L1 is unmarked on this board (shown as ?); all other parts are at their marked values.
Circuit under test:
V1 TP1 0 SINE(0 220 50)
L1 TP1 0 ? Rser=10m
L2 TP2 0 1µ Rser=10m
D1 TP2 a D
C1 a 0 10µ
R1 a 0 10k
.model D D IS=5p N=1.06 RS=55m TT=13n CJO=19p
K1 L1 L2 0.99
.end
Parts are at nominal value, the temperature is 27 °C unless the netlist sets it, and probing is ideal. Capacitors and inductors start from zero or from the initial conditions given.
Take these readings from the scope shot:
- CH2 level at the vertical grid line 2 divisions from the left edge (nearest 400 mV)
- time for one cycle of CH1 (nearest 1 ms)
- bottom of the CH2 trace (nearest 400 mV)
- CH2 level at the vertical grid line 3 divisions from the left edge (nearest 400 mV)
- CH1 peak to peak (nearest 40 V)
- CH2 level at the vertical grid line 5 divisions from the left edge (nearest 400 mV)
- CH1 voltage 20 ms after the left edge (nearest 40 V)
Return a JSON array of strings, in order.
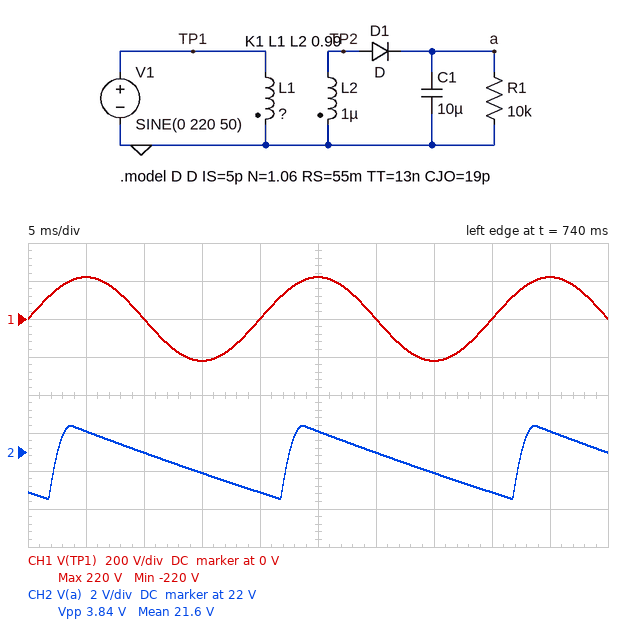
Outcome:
["22.0 V", "20 ms", "19.6 V", "20.8 V", "440 V", "23.2 V", "0 V"]
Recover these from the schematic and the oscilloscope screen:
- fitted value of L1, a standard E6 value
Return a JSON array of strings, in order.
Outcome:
["68 µH"]
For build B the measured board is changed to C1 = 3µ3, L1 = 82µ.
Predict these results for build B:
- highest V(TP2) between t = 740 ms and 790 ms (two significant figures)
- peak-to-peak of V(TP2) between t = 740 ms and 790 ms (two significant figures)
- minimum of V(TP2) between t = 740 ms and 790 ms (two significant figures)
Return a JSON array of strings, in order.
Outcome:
["22 V", "45 V", "-22 V"]
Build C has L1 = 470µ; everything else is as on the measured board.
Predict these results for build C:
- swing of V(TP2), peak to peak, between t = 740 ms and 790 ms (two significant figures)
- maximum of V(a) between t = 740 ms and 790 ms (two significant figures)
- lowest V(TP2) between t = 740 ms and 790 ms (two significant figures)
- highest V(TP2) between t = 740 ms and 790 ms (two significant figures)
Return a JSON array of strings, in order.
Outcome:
["20 V", "9.5 V", "-10 V", "10 V"]
